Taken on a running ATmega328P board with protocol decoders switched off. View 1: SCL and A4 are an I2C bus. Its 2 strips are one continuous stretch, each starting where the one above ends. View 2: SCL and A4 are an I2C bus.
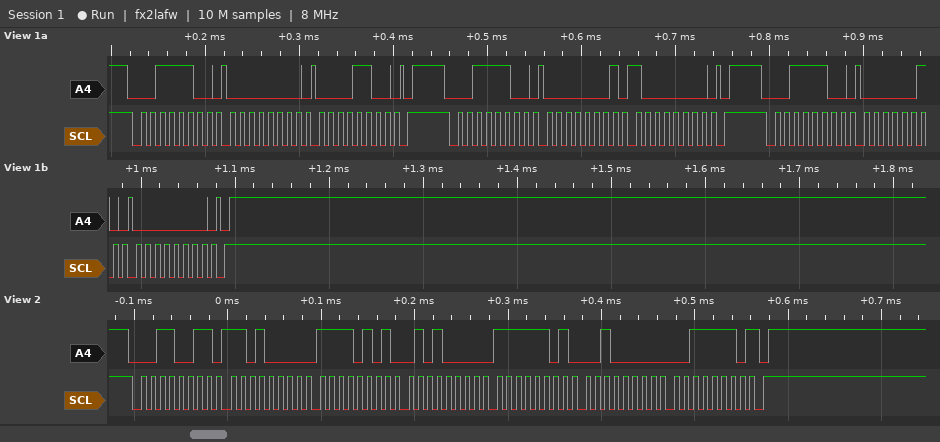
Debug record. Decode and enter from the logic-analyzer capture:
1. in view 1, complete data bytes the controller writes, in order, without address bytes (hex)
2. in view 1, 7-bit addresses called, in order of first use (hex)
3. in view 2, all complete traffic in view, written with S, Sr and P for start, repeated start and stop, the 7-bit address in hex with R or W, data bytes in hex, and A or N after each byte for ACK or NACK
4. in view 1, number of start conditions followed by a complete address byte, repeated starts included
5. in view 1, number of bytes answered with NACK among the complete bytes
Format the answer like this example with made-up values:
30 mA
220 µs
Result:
00 0C 01 80 02 00
0x1E
S 19R A D0 A F5 A 50 A FD A 20 A 3E N P
3
0
